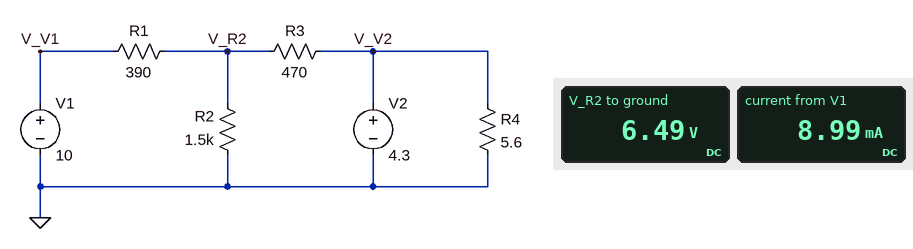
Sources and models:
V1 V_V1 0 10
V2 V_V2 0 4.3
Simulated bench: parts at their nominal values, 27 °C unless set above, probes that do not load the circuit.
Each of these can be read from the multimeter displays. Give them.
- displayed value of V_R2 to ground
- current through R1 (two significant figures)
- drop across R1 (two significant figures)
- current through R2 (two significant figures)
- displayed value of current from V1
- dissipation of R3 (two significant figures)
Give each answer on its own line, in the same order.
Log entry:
6.49 V
9.0 mA
3.5 V
4.3 mA
8.99 mA
10 mW
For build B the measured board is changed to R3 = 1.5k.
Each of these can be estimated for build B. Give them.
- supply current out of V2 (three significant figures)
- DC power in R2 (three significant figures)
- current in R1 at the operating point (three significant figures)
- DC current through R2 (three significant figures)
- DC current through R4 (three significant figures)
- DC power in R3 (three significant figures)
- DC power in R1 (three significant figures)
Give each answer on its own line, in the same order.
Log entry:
766 mA
35.7 mW
6.89 mA
4.88 mA
768 mA
6.06 mW
18.5 mW
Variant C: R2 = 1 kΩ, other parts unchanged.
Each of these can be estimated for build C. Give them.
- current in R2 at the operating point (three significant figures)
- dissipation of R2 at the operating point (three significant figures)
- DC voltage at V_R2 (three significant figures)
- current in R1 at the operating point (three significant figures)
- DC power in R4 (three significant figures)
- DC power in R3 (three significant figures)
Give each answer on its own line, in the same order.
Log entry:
6.11 mA
37.4 mW
6.11 V
9.97 mA
3.30 W
6.99 mW
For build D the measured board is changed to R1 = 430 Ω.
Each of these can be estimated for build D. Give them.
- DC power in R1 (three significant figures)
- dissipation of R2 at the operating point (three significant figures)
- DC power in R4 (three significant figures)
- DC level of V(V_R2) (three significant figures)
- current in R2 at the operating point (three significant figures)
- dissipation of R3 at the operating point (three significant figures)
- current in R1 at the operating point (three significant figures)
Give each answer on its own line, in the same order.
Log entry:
31.3 mW
26.7 mW
3.30 W
6.33 V
4.22 mA
8.76 mW
8.54 mA
